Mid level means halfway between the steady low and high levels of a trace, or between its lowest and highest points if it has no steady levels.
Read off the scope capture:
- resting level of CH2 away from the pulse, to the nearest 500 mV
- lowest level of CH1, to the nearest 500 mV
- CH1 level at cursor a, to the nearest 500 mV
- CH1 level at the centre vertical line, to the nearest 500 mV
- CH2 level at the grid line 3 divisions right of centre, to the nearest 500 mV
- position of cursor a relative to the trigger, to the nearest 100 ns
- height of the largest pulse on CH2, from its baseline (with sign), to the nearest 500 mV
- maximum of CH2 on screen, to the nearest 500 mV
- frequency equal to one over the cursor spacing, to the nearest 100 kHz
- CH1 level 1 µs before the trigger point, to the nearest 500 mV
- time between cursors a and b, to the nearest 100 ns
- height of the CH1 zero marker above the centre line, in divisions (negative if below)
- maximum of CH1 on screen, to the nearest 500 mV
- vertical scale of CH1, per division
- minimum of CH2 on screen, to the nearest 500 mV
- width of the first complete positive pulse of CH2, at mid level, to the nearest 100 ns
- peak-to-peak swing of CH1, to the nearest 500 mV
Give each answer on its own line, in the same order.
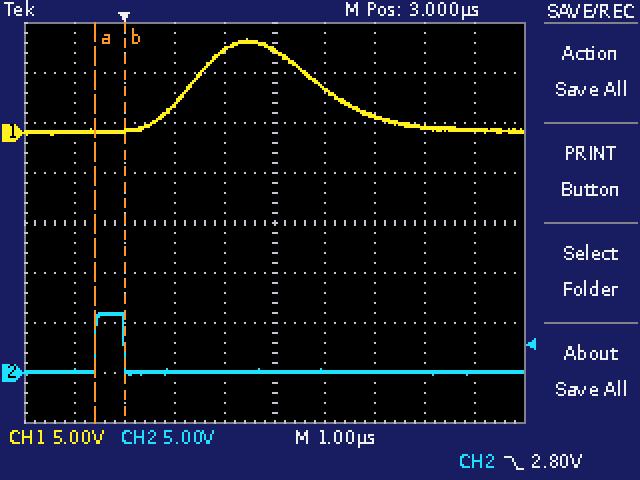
0.0 V
0.0 V
0.0 V
8.5 V
0.0 V
-600 ns
+6.0 V
6.0 V
1.7 MHz
0.0 V
600 ns
+1.8 div
9.5 V
5 V
0.0 V
600 ns
9.5 V
